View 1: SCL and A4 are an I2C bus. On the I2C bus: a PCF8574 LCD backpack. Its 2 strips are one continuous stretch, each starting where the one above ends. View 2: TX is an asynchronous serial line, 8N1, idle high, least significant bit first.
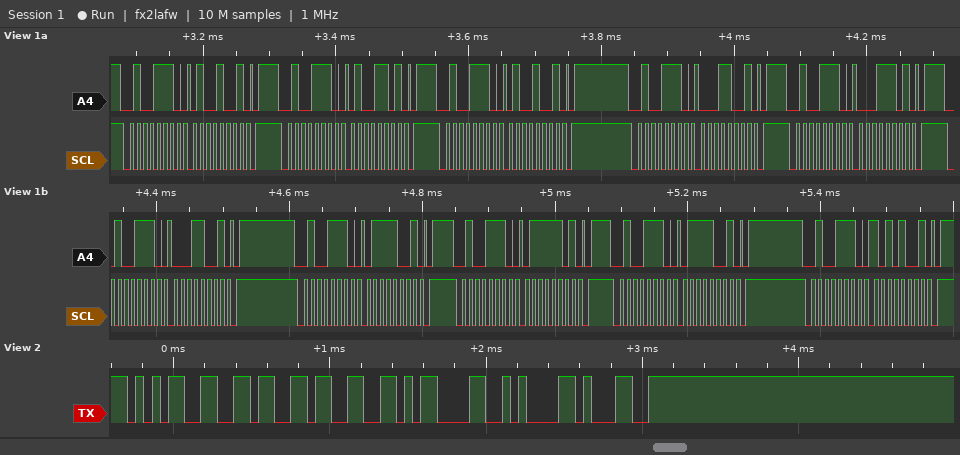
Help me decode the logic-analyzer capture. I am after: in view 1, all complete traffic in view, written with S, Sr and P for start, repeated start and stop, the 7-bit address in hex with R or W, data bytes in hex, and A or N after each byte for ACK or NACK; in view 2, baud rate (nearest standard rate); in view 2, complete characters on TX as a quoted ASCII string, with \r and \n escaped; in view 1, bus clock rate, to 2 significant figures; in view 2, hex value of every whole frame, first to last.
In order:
S 27W A 49 A P S 27W A 4D A P S 27W A 49 A P S 27W A 19 A P S 27W A 1D A P S 27W A 19 A P S 27W A 79 A P S 27W A 7D A P S 27W A 79 A P S 27W A A9 A P
19200 baud
"563\r\n1"
100 kHz
0x35 0x36 0x33 0x0D 0x0A 0x31
